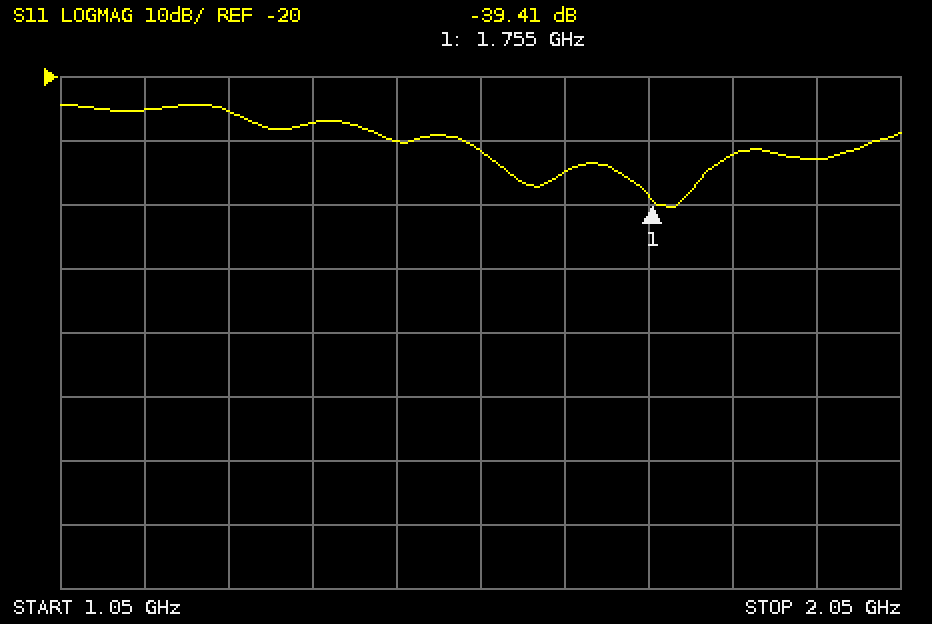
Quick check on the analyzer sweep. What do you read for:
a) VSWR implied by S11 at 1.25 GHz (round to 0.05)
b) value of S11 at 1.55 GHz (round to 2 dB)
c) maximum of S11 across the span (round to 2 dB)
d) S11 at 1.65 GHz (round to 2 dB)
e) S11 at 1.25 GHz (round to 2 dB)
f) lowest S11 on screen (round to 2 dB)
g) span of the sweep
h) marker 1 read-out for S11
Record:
1.10
-32 dB
-24 dB
-34 dB
-26 dB
-40 dB
1 GHz
-39.41 dB
